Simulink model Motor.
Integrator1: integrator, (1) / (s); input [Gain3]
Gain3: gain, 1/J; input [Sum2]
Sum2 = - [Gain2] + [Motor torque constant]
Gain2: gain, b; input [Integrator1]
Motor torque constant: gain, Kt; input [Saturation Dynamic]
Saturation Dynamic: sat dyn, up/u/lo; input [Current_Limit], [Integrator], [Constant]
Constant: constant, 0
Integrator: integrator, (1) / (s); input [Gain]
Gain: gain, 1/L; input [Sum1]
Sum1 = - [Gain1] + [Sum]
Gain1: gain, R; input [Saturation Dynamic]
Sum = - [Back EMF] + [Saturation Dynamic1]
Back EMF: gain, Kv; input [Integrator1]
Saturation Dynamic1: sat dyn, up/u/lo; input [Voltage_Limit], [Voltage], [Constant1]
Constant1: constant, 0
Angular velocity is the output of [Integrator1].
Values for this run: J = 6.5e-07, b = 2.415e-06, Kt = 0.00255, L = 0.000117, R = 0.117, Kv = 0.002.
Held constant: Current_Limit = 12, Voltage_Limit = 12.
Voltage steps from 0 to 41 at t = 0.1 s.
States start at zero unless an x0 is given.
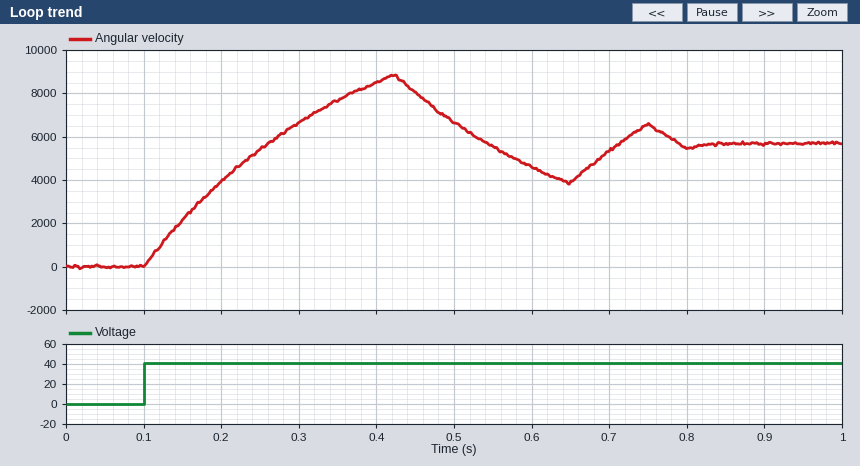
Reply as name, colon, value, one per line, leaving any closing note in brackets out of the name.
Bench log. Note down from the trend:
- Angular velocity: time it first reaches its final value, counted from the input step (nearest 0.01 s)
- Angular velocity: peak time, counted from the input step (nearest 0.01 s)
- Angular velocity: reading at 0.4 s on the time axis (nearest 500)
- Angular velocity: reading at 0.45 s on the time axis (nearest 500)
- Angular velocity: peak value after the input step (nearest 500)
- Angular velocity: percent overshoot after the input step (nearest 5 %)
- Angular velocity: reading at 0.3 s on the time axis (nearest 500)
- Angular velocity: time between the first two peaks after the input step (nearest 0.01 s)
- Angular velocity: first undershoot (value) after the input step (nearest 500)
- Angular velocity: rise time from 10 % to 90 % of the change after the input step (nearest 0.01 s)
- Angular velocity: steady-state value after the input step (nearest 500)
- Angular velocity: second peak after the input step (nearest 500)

Angular velocity: time it first reaches its final value, counted from the input step: 0.16 s
Angular velocity: peak time, counted from the input step: 0.32 s
Angular velocity: reading at 0.4 s on the time axis: 8500
Angular velocity: reading at 0.45 s on the time axis: 8000
Angular velocity: peak value after the input step: 9000
Angular velocity: percent overshoot after the input step: 55 %
Angular velocity: reading at 0.3 s on the time axis: 6500
Angular velocity: time between the first two peaks after the input step: 0.33 s
Angular velocity: first undershoot (value) after the input step: 4000
Angular velocity: rise time from 10 % to 90 % of the change after the input step: 0.13 s
Angular velocity: steady-state value after the input step: 5500
Angular velocity: second peak after the input step: 6500
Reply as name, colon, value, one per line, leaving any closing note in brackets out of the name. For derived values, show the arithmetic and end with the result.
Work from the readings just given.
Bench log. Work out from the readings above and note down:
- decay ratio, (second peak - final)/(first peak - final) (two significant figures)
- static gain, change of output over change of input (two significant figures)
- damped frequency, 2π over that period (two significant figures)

decay ratio, (second peak - final)/(first peak - final): (6500 - 5500) / (9000 - 5500) = 0.29
static gain, change of output over change of input: (5500 - 0) / (41 - 0) = 130
damped frequency, 2π over that period: 2π / 0.33 = 19 rad/s
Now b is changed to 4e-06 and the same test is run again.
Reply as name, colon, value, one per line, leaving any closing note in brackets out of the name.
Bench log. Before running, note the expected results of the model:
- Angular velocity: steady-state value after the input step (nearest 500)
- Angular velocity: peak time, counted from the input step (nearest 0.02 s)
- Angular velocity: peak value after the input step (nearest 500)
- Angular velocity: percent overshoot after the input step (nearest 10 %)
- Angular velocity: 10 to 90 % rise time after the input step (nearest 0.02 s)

Angular velocity: steady-state value after the input step: 5500
Angular velocity: peak time, counted from the input step: 0.50 s
Angular velocity: peak value after the input step: 7500
Angular velocity: percent overshoot after the input step: 30 %
Angular velocity: 10 to 90 % rise time after the input step: 0.16 s
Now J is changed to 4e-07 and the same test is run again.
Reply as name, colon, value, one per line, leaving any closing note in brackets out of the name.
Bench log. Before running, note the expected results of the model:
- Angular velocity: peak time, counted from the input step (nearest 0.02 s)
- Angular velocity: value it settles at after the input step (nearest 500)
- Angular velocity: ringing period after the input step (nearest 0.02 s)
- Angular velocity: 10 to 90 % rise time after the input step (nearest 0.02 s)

Angular velocity: peak time, counted from the input step: 0.20 s
Angular velocity: value it settles at after the input step: 5500
Angular velocity: ringing period after the input step: 0.20 s
Angular velocity: 10 to 90 % rise time after the input step: 0.08 s
